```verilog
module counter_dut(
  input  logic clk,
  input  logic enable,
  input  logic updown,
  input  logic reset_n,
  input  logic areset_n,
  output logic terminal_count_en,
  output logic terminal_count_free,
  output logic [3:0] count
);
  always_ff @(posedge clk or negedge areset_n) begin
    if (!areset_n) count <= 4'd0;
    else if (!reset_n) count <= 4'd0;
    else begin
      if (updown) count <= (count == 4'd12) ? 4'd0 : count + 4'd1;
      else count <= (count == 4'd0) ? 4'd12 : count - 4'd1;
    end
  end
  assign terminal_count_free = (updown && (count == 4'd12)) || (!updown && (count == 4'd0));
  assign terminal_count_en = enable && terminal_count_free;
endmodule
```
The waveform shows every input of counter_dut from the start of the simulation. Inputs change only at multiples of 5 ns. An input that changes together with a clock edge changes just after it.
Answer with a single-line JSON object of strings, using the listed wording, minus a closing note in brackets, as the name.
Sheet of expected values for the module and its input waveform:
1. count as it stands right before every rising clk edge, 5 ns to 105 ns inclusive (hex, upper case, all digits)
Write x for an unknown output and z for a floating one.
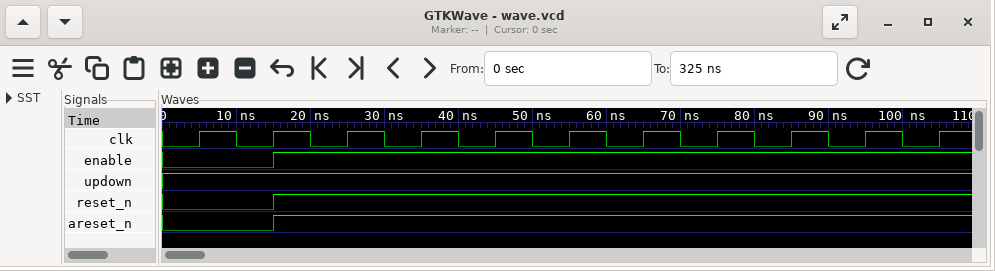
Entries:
{"count as it stands right before every rising clk edge, 5 ns to 105 ns inclusive": "0, 0, 0, 1, 2, 3, 4, 5, 6, 7, 8"}
